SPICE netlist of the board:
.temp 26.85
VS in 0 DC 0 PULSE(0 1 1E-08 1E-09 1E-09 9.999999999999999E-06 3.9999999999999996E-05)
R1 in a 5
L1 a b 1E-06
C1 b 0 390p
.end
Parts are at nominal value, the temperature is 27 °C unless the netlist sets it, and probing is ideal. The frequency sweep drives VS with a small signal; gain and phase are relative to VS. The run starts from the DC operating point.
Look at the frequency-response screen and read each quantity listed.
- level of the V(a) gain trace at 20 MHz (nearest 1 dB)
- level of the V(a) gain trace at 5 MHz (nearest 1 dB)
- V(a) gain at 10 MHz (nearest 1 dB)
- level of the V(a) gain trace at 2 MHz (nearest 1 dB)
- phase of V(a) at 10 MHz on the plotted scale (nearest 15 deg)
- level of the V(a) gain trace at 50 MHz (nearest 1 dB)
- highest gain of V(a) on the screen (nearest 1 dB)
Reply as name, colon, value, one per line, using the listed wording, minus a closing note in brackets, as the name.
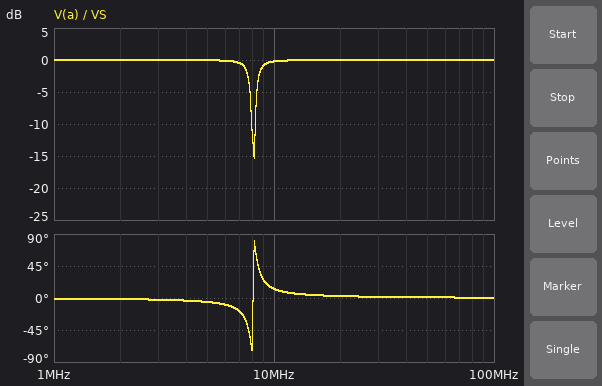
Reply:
level of the V(a) gain trace at 20 MHz: 0 dB
level of the V(a) gain trace at 5 MHz: 0 dB
V(a) gain at 10 MHz: 0 dB
level of the V(a) gain trace at 2 MHz: 0 dB
phase of V(a) at 10 MHz on the plotted scale: 15 deg
level of the V(a) gain trace at 50 MHz: 0 dB
highest gain of V(a) on the screen: 0 dB
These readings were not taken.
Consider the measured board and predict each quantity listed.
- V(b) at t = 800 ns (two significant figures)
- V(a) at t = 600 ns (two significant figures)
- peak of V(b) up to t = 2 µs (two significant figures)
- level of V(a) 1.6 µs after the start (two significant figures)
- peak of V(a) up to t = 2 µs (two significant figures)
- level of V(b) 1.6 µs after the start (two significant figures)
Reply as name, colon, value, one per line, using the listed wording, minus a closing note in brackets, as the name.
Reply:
V(b) at t = 800 ns: 1.1 V
V(a) at t = 600 ns: 1.0 V
peak of V(b) up to t = 2 µs: 1.9 V
level of V(a) 1.6 µs after the start: 1.0 V
peak of V(a) up to t = 2 µs: 1.1 V
level of V(b) 1.6 µs after the start: 1.0 V
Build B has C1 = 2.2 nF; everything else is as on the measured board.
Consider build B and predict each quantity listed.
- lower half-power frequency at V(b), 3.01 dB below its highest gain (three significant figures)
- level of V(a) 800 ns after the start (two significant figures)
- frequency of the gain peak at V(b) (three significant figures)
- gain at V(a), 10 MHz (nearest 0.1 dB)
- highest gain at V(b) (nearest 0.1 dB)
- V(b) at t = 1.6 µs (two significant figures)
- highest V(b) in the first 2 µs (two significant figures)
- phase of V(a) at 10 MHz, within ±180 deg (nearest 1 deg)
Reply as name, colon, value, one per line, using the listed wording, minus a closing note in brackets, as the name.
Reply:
lower half-power frequency at V(b), 3.01 dB below its highest gain: 2.92 MHz
level of V(a) 800 ns after the start: 1.0 V
frequency of the gain peak at V(b): 3.35 MHz
gain at V(a), 10 MHz: 0 dB
highest gain at V(b): 12.7 dB
V(b) at t = 1.6 µs: 1.0 V
highest V(b) in the first 2 µs: 1.7 V
phase of V(a) at 10 MHz, within ±180 deg: 5 deg
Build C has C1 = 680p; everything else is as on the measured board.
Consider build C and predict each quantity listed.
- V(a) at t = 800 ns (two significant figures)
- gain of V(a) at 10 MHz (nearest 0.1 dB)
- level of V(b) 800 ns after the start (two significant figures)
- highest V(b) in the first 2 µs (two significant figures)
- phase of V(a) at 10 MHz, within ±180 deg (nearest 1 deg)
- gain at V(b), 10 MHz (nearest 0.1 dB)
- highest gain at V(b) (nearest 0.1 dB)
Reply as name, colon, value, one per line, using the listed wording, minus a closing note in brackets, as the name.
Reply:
V(a) at t = 800 ns: 1.0 V
gain of V(a) at 10 MHz: -0.1 dB
level of V(b) 800 ns after the start: 960 mV
highest V(b) in the first 2 µs: 1.8 V
phase of V(a) at 10 MHz, within ±180 deg: 7 deg
gain at V(b), 10 MHz: -4.6 dB
highest gain at V(b): 17.7 dB
